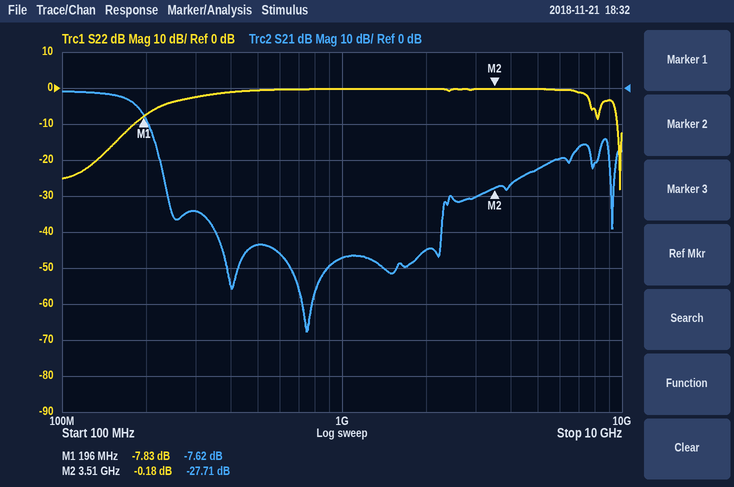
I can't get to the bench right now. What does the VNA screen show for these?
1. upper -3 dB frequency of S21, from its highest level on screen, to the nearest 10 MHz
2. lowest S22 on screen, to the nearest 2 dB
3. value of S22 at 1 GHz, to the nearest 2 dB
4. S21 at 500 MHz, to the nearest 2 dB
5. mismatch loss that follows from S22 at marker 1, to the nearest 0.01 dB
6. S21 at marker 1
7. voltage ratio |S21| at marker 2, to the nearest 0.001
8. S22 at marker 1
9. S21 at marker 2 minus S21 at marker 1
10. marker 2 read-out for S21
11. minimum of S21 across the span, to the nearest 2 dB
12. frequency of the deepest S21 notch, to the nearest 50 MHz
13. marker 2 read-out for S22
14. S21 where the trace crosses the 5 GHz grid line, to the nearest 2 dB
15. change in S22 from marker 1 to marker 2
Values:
180 MHz
-28 dB
0 dB
-44 dB
0.78 dB
-7.62 dB
0.041
-7.83 dB
-20.09 dB
-27.71 dB
-68 dB
750 MHz
-0.18 dB
-22 dB
7.65 dB
